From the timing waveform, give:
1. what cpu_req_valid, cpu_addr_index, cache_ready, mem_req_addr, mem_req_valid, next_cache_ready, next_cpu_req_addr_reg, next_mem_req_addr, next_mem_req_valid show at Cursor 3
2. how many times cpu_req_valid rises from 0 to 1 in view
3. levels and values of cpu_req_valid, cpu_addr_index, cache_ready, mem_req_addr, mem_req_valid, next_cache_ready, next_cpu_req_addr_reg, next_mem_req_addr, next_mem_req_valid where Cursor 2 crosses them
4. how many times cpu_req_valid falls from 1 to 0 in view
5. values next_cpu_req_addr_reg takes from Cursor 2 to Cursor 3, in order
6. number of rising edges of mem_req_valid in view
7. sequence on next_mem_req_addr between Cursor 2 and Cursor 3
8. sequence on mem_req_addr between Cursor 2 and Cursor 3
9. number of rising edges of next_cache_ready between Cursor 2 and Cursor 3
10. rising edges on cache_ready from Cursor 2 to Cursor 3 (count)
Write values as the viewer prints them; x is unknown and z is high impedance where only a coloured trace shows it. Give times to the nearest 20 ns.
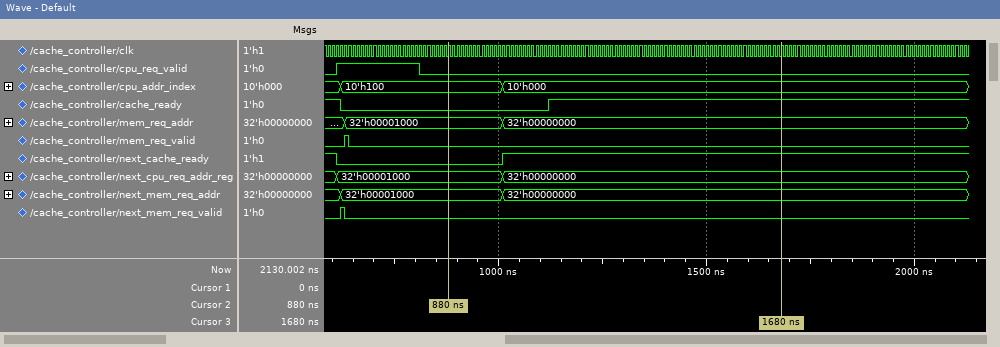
cpu_req_valid=0, cpu_addr_index=10'h000, cache_ready=1, mem_req_addr=32'h00000000, mem_req_valid=0, next_cache_ready=1, next_cpu_req_addr_reg=32'h00000000, next_mem_req_addr=32'h00000000, next_mem_req_valid=0
1
cpu_req_valid=0, cpu_addr_index=10'h100, cache_ready=0, mem_req_addr=32'h00001000, mem_req_valid=0, next_cache_ready=0, next_cpu_req_addr_reg=32'h00001000, next_mem_req_addr=32'h00001000, next_mem_req_valid=0
1
32'h00001000, 32'h00000000
1
32'h00001000, 32'h00000000
32'h00001000, 32'h00000000
1
1
